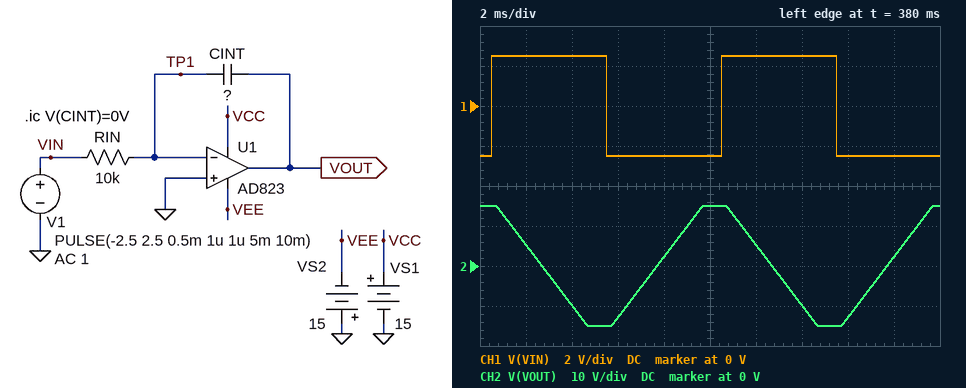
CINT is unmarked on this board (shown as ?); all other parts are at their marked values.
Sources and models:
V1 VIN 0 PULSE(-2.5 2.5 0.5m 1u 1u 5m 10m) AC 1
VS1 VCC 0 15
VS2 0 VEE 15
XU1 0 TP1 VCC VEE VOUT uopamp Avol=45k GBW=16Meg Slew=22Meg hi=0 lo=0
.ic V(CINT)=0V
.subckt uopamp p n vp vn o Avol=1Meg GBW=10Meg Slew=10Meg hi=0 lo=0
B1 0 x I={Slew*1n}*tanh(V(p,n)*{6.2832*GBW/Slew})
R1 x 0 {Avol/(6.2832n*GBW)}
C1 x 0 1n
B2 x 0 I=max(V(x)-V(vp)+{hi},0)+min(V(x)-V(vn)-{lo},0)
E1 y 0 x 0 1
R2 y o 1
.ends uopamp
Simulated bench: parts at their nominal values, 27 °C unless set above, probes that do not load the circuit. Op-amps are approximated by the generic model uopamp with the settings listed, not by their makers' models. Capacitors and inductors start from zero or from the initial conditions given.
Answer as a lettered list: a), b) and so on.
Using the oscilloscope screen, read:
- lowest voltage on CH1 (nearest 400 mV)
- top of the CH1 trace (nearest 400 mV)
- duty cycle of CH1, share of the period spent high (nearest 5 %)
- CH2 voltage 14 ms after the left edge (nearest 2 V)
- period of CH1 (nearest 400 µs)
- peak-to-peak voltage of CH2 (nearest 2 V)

a) -2.4 V
b) 2.4 V
c) 50 %
d) -10 V
e) 10.0 ms
f) 30 V
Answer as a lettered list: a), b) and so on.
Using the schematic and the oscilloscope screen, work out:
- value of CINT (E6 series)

a) 33 nF
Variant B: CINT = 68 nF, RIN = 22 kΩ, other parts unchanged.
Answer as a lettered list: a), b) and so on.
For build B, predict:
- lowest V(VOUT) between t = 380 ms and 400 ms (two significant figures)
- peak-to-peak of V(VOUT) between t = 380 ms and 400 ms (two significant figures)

a) -7.6 V
b) 8.4 V
